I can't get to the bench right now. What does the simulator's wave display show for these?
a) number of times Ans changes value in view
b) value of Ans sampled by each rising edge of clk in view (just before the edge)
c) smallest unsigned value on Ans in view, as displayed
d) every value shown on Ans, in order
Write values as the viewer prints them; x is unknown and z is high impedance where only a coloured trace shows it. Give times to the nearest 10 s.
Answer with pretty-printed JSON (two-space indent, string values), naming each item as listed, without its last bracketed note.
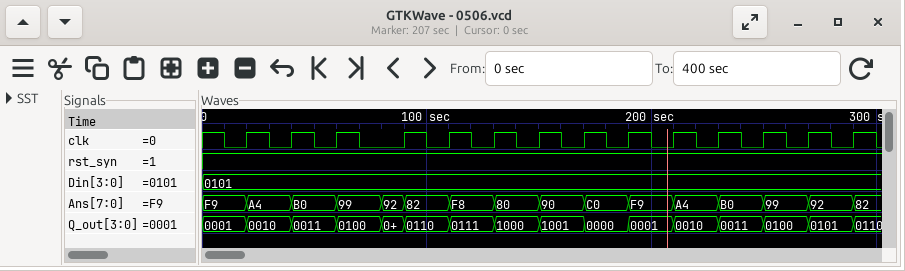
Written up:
{
  "number of times Ans changes value in view": "15",
  "value of Ans sampled by each rising edge of clk in view": "F9, A4, B0, 92, 82, F8, 80, 90, C0, F9, A4, B0, 99, 92",
  "smallest unsigned value on Ans in view, as displayed": "80",
  "every value shown on Ans, in order": "F9, A4, B0, 99, 92, 82, F8, 80, 90, C0, F9, A4, B0, 99, 92, 82"
}
